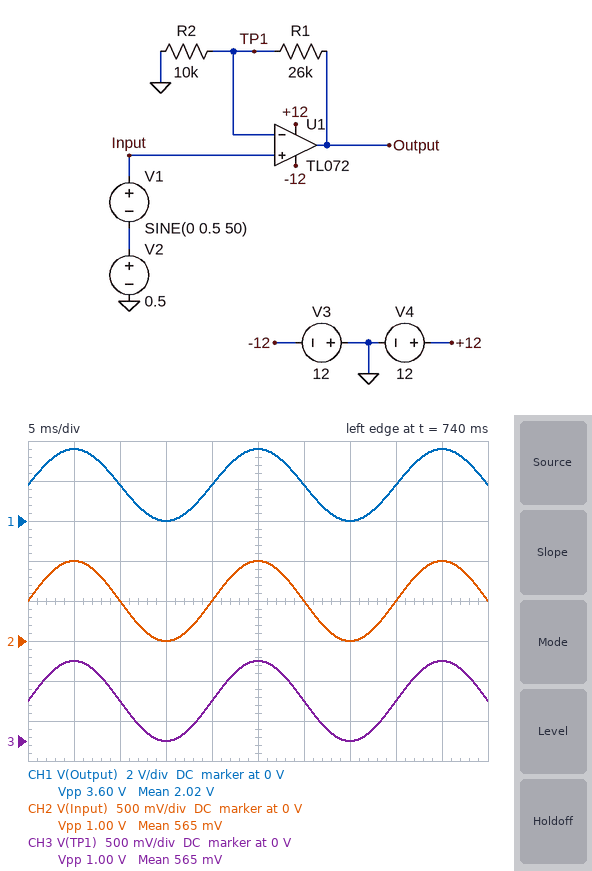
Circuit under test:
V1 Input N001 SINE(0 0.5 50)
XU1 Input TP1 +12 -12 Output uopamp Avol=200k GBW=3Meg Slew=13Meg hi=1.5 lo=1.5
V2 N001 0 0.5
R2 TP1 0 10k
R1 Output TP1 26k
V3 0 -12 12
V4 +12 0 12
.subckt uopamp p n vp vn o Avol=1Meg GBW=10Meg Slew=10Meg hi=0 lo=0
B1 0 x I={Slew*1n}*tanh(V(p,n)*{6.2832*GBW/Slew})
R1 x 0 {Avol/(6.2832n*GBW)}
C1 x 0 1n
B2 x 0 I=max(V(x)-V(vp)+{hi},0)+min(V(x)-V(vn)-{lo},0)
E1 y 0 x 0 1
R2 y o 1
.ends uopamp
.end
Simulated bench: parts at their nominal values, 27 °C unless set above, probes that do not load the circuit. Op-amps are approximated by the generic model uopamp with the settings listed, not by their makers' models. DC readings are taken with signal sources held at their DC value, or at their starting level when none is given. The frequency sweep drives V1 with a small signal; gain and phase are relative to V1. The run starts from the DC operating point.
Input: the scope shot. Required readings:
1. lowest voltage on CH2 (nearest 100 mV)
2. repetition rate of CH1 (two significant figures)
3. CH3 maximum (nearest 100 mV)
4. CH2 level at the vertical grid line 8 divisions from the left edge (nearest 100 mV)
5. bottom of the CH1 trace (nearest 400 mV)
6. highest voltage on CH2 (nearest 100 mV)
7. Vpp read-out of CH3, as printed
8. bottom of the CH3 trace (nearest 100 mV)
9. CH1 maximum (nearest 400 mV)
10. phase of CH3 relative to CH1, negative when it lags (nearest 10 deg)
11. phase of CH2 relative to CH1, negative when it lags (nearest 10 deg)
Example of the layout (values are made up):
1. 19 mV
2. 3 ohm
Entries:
1. 0 V
2. 50 Hz
3. 1.0 V
4. 500 mV
5. 0 V
6. 1.0 V
7. 1.00 V
8. 0 V
9. 3.6 V
10. 0 deg
11. 0 deg
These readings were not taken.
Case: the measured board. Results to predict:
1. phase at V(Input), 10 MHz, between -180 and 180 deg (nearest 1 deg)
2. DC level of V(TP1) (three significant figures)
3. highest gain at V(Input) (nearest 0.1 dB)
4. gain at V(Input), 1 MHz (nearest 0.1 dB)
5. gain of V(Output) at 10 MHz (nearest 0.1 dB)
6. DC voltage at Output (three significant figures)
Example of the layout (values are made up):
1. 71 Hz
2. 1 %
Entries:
1. 0 deg
2. 500 mV
3. 0 dB
4. 0 dB
5. -10.5 dB
6. 1.80 V
